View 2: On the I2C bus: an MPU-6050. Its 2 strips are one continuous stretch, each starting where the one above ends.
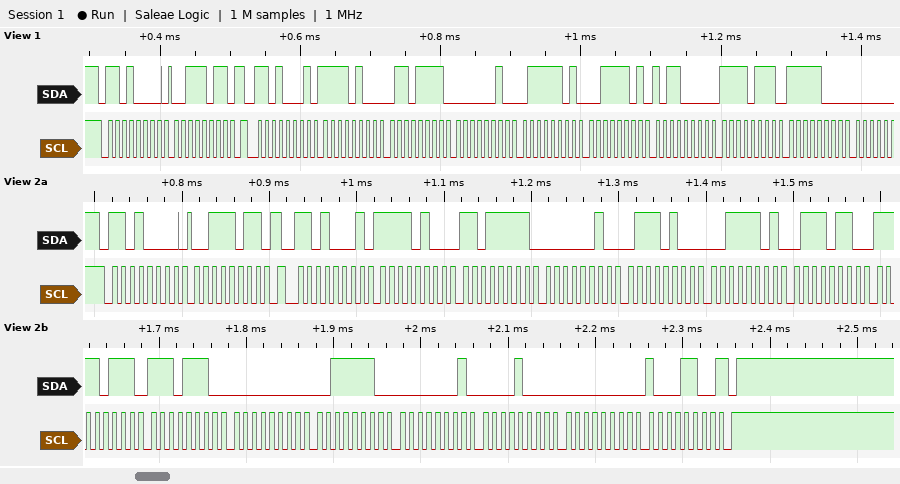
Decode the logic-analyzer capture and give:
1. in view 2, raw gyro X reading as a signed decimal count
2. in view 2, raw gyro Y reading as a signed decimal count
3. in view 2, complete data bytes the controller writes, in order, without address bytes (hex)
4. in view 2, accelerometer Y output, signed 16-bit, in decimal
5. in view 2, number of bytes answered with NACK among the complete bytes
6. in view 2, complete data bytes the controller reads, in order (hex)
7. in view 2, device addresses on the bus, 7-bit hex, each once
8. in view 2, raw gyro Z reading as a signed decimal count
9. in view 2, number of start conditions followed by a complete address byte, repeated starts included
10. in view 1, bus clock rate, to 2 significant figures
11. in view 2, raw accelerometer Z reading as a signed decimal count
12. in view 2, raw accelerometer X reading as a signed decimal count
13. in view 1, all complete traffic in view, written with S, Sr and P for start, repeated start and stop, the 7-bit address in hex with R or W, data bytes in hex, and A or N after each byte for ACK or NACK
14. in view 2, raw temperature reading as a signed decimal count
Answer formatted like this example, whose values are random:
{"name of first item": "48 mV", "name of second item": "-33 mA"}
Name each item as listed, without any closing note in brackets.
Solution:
{"in view 2, raw gyro X reading as a signed decimal count": "62", "in view 2, raw gyro Y reading as a signed decimal count": "264", "in view 2, complete data bytes the controller writes, in order, without address bytes": "3B", "in view 2, accelerometer Y output, signed 16-bit, in decimal": "628", "in view 2, number of bytes answered with NACK among the complete bytes": "1", "in view 2, complete data bytes the controller reads, in order": "F4 DF 02 74 3D 76 F7 EE 00 3E 01 08 00 8C", "in view 2, device addresses on the bus, 7-bit hex, each once": "0x68", "in view 2, raw gyro Z reading as a signed decimal count": "140", "in view 2, number of start conditions followed by a complete address byte, repeated starts included": "2", "in view 1, bus clock rate, to 2 significant figures": "100 kHz", "in view 2, raw accelerometer Z reading as a signed decimal count": "15734", "in view 2, raw accelerometer X reading as a signed decimal count": "-2849", "in view 1, all complete traffic in view, written with S, Sr and P for start, repeated start and stop, the 7-bit address in hex with R or W, data bytes in hex, and A or N after each byte for ACK or NACK": "S 68W A 3B A Sr 68R A F4 A 6F A 02 A 7D A 3D A B0 A F7 A F8 A", "in view 2, raw temperature reading as a signed decimal count": "-2066"}
